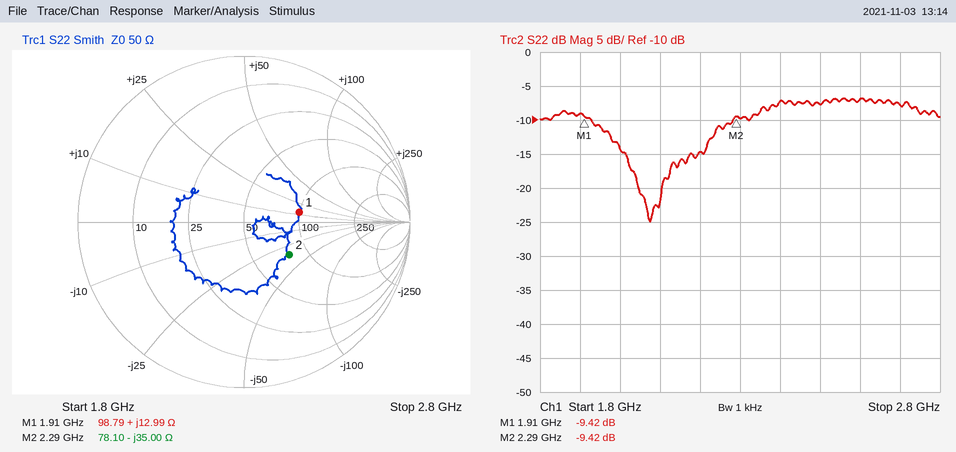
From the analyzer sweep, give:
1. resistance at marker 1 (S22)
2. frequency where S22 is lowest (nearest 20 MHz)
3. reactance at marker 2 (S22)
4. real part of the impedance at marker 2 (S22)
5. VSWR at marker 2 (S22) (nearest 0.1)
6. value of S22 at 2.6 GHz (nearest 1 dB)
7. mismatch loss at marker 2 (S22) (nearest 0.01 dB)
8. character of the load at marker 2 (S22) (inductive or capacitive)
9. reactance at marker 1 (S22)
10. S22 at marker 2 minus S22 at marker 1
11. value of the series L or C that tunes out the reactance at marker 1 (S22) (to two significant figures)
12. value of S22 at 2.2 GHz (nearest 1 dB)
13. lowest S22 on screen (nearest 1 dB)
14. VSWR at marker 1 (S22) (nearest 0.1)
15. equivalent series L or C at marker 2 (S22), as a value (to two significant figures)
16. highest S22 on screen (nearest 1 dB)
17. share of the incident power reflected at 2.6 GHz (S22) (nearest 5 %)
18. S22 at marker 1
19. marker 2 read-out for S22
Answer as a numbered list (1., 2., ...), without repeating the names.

1. 98.79 Ω
2. 2.08 GHz
3. -35.00 Ω
4. 78.10 Ω
5. 2.0
6. -7 dB
7. 0.53 dB
8. capacitive
9. +12.99 Ω
10. 0.00 dB
11. 6.4 pF
12. -15 dB
13. -25 dB
14. 2.0
15. 2.0 pF
16. -7 dB
17. 20 %
18. -9.42 dB
19. -9.42 dB
